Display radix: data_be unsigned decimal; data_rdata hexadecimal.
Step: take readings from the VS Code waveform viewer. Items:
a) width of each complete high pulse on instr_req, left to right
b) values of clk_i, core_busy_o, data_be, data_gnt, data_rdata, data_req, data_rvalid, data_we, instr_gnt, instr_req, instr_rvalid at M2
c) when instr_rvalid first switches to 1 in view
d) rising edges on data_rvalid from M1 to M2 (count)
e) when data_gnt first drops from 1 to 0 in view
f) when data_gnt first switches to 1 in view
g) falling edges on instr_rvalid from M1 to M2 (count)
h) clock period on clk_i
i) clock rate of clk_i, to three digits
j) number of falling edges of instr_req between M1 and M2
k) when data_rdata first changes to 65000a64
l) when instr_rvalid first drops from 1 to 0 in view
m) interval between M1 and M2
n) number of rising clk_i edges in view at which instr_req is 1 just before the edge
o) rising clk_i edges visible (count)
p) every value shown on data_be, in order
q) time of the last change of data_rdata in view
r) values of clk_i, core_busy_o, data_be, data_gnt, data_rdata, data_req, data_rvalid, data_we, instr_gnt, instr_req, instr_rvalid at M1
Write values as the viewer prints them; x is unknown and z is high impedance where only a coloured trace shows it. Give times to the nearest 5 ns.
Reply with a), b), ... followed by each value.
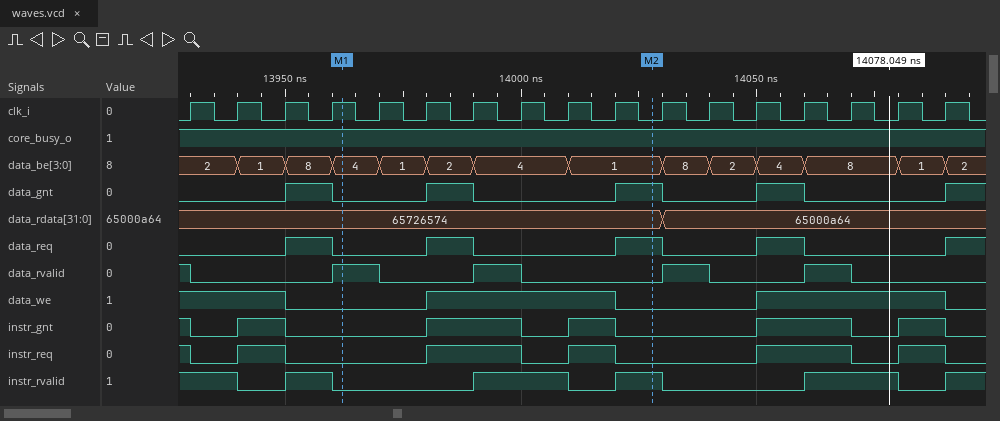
a) 10 ns, 20 ns, 10 ns, 20 ns, 10 ns
b) clk_i=0, core_busy_o=1, data_be=1, data_gnt=1, data_rdata=65726574, data_req=1, data_rvalid=0, data_we=0, instr_gnt=0, instr_req=0, instr_rvalid=1
c) 13950 ns
d) 1
e) 13960 ns
f) 13950 ns
g) 1
h) 10 ns
i) 100 MHz
j) 2
k) 14030 ns
l) 13940 ns
m) 65 ns
n) 8
o) 17
p) 2, 1, 8, 4, 1, 2, 4, 1, 8, 2, 4, 8, 1, 2
q) 14030 ns
r) clk_i=1, core_busy_o=1, data_be=4, data_gnt=0, data_rdata=65726574, data_req=0, data_rvalid=1, data_we=0, instr_gnt=0, instr_req=0, instr_rvalid=0
